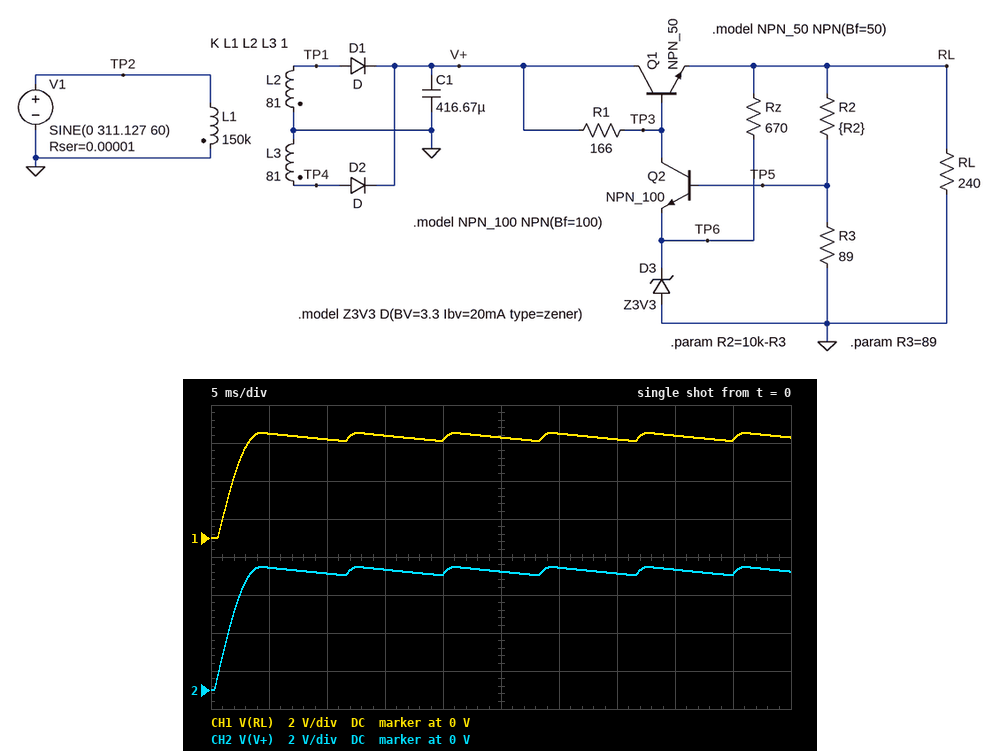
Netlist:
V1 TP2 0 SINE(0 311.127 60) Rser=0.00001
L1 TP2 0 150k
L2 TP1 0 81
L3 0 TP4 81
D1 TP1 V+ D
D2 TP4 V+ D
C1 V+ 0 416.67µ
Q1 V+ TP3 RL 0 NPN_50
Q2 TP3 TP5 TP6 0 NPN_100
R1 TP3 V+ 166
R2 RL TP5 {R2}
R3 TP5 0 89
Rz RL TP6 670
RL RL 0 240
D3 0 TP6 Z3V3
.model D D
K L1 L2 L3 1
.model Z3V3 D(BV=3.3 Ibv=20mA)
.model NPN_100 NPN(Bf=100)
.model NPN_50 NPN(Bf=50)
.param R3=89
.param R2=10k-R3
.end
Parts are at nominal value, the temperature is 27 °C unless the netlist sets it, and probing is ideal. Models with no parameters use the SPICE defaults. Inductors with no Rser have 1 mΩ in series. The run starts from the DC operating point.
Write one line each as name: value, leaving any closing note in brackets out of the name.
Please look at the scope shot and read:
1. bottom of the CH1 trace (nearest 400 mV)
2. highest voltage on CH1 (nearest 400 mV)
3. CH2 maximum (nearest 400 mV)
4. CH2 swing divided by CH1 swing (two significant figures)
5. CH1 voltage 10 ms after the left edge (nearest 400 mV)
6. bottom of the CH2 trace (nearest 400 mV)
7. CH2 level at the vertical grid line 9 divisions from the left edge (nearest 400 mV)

bottom of the CH1 trace: 0 V
highest voltage on CH1: 5.6 V
CH2 maximum: 6.4 V
CH2 swing divided by CH1 swing: 1.2
CH1 voltage 10 ms after the left edge: 5.2 V
bottom of the CH2 trace: 0 V
CH2 level at the vertical grid line 9 divisions from the left edge: 6.0 V
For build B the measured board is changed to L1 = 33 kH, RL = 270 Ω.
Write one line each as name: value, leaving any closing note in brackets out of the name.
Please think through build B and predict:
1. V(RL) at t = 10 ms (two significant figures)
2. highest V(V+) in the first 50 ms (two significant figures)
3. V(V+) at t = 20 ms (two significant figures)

V(RL) at t = 10 ms: 13 V
highest V(V+) in the first 50 ms: 15 V
V(V+) at t = 20 ms: 14 V
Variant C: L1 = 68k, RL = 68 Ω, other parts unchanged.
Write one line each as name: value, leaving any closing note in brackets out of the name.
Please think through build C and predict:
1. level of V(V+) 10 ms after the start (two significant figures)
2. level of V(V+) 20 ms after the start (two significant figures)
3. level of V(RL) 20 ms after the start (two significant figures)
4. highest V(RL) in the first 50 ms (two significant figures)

level of V(V+) 10 ms after the start: 8.3 V
level of V(V+) 20 ms after the start: 9.4 V
level of V(RL) 20 ms after the start: 8.1 V
highest V(RL) in the first 50 ms: 8.6 V
